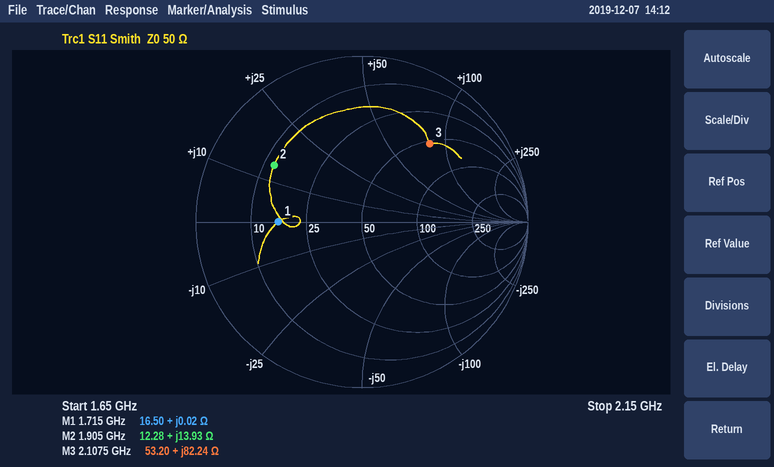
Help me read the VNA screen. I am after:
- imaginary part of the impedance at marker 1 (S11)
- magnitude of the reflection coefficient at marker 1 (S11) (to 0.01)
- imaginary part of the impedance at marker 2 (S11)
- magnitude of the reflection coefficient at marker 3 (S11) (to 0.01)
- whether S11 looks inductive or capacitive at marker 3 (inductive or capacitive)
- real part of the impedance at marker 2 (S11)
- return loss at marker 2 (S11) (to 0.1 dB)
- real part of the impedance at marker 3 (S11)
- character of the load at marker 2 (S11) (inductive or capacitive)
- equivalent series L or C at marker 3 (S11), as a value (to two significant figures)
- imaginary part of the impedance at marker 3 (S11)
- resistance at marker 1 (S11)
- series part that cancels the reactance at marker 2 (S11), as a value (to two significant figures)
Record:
+0.02 Ω
0.50
+13.93 Ω
0.62
inductive
12.28 Ω
4.0 dB
53.20 Ω
inductive
6.2 nH
+82.24 Ω
16.50 Ω
6.0 pF
